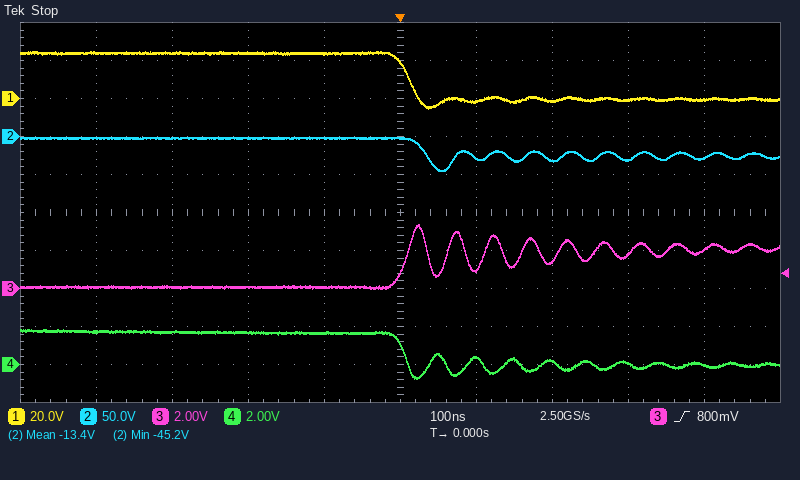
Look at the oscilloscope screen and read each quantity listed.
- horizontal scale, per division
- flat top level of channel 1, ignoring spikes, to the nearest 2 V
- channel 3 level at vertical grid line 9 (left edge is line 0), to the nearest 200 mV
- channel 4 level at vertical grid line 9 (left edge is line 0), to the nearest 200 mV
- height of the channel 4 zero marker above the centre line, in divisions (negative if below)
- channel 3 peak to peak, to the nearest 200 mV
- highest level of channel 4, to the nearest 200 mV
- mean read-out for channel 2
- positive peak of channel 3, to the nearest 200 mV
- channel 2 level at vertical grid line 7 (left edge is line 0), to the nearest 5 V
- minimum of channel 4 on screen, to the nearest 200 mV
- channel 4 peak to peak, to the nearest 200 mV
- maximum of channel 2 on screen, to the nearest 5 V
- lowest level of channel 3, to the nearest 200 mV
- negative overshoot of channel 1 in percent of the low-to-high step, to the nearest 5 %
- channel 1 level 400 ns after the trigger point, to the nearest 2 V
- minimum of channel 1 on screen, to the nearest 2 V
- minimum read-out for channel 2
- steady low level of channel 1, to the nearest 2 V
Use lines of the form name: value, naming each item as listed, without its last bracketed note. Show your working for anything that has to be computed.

horizontal scale, per division: 100 ns
flat top level of channel 1, ignoring spikes, to the nearest 2 V: 24 V
channel 3 level at vertical grid line 9 (left edge is line 0), to the nearest 200 mV: 2.0 V
channel 4 level at vertical grid line 9 (left edge is line 0), to the nearest 200 mV: 0.0 V
height of the channel 4 zero marker above the centre line, in divisions: -4.0 div
channel 3 peak to peak, to the nearest 200 mV: 3.4 V − (0.0 V) = 3.4 V
highest level of channel 4, to the nearest 200 mV: 1.8 V
mean read-out for channel 2: -13.4 V
positive peak of channel 3, to the nearest 200 mV: 3.4 V
channel 2 level at vertical grid line 7 (left edge is line 0), to the nearest 5 V: -30 V
minimum of channel 4 on screen, to the nearest 200 mV: -800 mV
channel 4 peak to peak, to the nearest 200 mV: 1.8 V − (-800 mV) = 2.6 V
maximum of channel 2 on screen, to the nearest 5 V: 0 V
lowest level of channel 3, to the nearest 200 mV: 0.0 V
negative overshoot of channel 1 in percent of the low-to-high step, to the nearest 5 %: 20 %
channel 1 level 400 ns after the trigger point, to the nearest 2 V: 0 V
minimum of channel 1 on screen, to the nearest 2 V: -6 V
minimum read-out for channel 2: -45.2 V
steady low level of channel 1, to the nearest 2 V: 0 V
